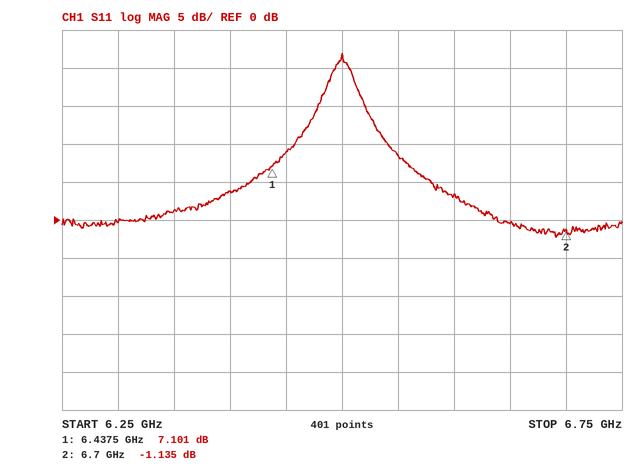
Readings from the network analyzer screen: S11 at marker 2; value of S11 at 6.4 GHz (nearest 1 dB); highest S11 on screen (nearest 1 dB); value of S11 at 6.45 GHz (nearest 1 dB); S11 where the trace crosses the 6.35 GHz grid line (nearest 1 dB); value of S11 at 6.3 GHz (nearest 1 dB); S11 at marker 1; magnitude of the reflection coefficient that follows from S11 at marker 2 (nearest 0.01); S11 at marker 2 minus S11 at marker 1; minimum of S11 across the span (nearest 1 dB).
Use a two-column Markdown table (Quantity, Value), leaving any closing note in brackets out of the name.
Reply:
| Quantity | Value |
|---|---|
| S11 at marker 2 | -1.135 dB |
| value of S11 at 6.4 GHz | 4 dB |
| highest S11 on screen | 22 dB |
| value of S11 at 6.45 GHz | 9 dB |
| S11 where the trace crosses the 6.35 GHz grid line | 1 dB |
| value of S11 at 6.3 GHz | 0 dB |
| S11 at marker 1 | 7.101 dB |
| magnitude of the reflection coefficient that follows from S11 at marker 2 | 0.88 |
| S11 at marker 2 minus S11 at marker 1 | -8.236 dB |
| minimum of S11 across the span | -2 dB |
